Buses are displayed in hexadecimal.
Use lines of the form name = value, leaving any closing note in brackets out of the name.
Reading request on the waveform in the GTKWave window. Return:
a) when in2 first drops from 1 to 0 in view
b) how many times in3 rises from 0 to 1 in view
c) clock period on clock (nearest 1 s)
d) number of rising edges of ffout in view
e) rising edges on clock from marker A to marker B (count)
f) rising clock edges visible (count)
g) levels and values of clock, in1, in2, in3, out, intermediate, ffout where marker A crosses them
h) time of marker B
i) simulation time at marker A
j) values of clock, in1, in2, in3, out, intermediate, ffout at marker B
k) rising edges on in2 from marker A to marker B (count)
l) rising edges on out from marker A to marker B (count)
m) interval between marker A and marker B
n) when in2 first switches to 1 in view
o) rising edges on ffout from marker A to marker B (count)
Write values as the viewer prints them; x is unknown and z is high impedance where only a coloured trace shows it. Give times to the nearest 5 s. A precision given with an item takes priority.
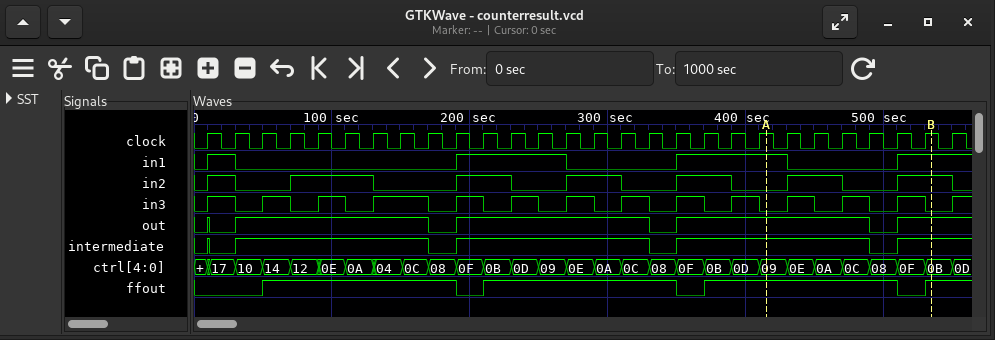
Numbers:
when in2 first drops from 1 to 0 in view = 30 s
how many times in3 rises from 0 to 1 in view = 14
clock period on clock = 20 s
number of rising edges of ffout in view = 4
rising edges on clock from marker A to marker B = 6
rising clock edges visible = 28
levels and values of clock, in1, in2, in3, out, intermediate, ffout where marker A crosses them = clock=1, in1=1, in2=0, in3=0, out=1, intermediate=1, ffout=1
time of marker B = 535 s
simulation time at marker A = 415 s
values of clock, in1, in2, in3, out, intermediate, ffout at marker B = clock=1, in1=1, in2=1, in3=0, out=1, intermediate=1, ffout=1
rising edges on in2 from marker A to marker B = 2
rising edges on out from marker A to marker B = 1
interval between marker A and marker B = 120 s
when in2 first switches to 1 in view = 10 s
rising edges on ffout from marker A to marker B = 1
